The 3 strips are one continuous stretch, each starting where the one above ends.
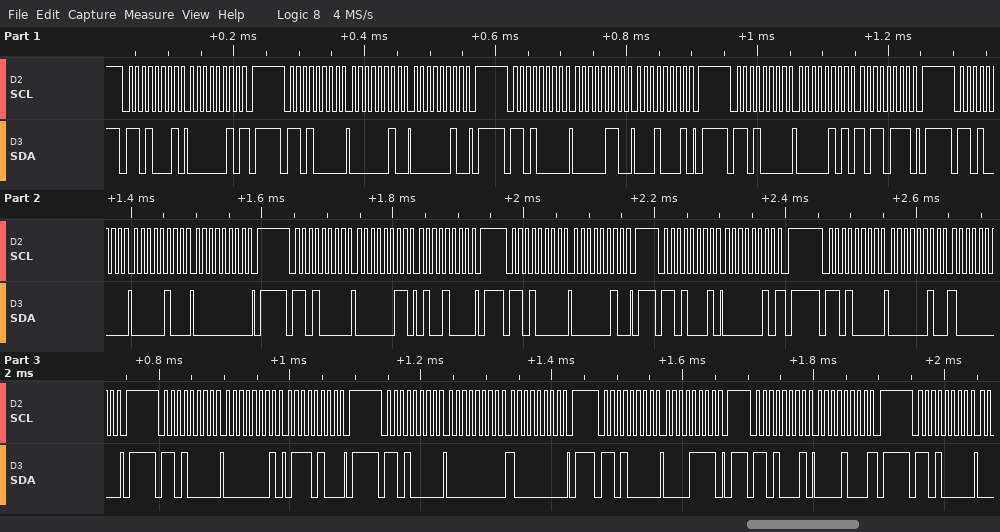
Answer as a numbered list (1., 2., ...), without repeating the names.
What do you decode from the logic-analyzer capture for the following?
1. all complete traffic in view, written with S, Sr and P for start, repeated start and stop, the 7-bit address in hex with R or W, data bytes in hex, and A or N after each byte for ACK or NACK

1. S 68R A 02 N P S 68W A 02 A 02 A P S 68W A 06 A 11 A P S 68W A 05 A B7 A P S 68W A 04 A 00 A P S 68W A 03 A 48 A P S 68W A 02 A P S 68R A 02 N P S 68W A 02 A 80 A P S 68W A 01 A 74 A P S 68W A 00 A 80 A P S 68W A 0F A P S 68R A 08 N P S 68W A
